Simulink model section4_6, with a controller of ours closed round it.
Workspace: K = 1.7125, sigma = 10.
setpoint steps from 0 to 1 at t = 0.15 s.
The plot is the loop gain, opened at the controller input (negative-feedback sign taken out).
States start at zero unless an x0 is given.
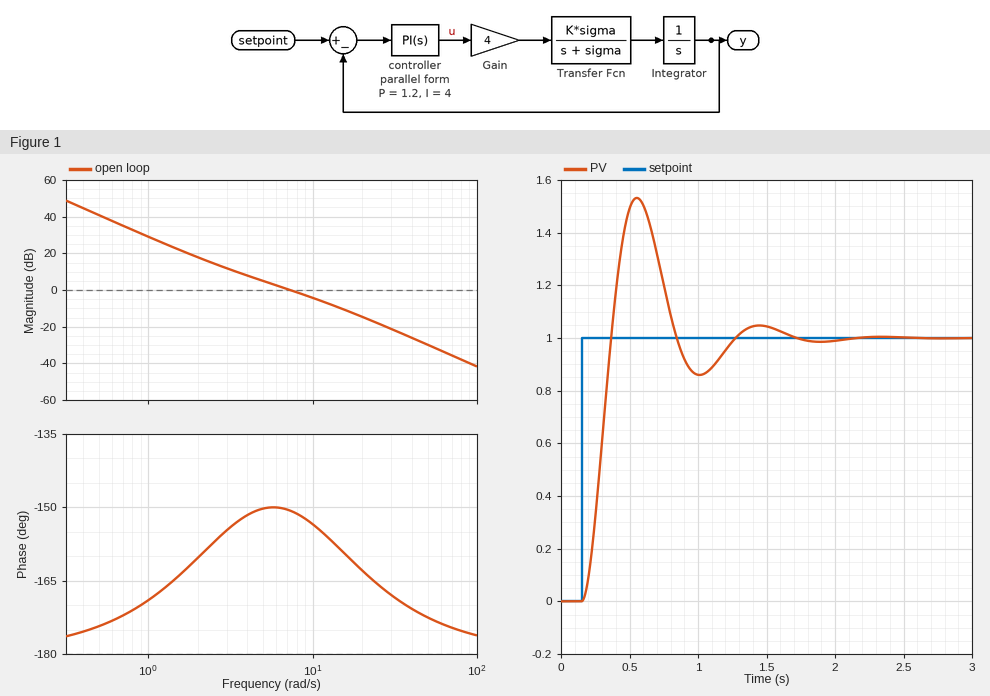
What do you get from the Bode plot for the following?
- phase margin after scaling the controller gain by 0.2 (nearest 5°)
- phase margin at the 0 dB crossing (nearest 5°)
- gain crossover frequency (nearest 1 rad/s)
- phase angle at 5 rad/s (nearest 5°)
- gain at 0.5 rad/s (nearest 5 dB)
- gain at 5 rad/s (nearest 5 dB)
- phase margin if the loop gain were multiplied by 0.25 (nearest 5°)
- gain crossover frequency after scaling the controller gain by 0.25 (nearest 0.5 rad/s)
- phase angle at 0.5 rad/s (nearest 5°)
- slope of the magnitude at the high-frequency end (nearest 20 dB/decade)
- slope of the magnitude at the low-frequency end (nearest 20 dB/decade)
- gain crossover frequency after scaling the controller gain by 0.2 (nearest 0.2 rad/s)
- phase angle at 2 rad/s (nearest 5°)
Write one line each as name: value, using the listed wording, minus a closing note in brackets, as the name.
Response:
phase margin after scaling the controller gain by 0.2: 25°
phase margin at the 0 dB crossing: 30°
gain crossover frequency: 7 rad/s
phase angle at 5 rad/s: -150°
gain at 0.5 rad/s: 40 dB
gain at 5 rad/s: 5 dB
phase margin if the loop gain were multiplied by 0.25: 25°
gain crossover frequency after scaling the controller gain by 0.25: 3.0 rad/s
phase angle at 0.5 rad/s: -175°
slope of the magnitude at the high-frequency end: -40 dB/decade
slope of the magnitude at the low-frequency end: -40 dB/decade
gain crossover frequency after scaling the controller gain by 0.2: 2.6 rad/s
phase angle at 2 rad/s: -160°
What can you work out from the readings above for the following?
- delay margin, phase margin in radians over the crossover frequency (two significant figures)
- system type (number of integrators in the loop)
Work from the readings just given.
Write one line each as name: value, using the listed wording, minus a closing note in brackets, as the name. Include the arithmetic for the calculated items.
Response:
delay margin, phase margin in radians over the crossover frequency: 30 × π / 180 / 7 = 0.075 s
system type: 2
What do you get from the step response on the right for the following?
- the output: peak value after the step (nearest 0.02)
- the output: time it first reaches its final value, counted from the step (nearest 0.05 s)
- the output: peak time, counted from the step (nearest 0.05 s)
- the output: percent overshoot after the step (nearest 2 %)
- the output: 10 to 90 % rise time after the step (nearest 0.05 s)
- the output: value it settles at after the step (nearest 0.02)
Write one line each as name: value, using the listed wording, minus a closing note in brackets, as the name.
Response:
the output: peak value after the step: 1.54
the output: time it first reaches its final value, counted from the step: 0.20 s
the output: peak time, counted from the step: 0.40 s
the output: percent overshoot after the step: 54 %
the output: 10 to 90 % rise time after the step: 0.15 s
the output: value it settles at after the step: 1.00
